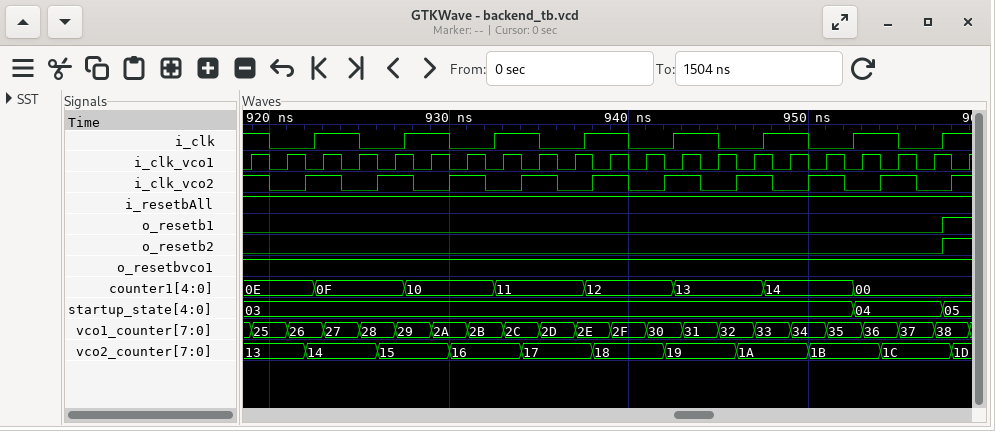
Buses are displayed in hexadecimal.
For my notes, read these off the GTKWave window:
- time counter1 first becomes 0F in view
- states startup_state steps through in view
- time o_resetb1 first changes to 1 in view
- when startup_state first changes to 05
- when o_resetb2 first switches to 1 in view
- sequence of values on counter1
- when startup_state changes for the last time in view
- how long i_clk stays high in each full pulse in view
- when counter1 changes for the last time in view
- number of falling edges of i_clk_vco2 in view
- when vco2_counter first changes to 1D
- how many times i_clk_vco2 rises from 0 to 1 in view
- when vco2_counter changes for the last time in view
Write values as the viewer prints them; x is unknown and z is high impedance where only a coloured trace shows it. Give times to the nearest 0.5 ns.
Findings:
922.5 ns
03, 04, 05
957.5 ns
957.5 ns
957.5 ns
0E, 0F, 10, 11, 12, 13, 14, 00
957.5 ns
2.5 ns, 2.5 ns, 2.5 ns, 2.5 ns, 2.5 ns, 2.5 ns, 2.5 ns
952.5 ns
10
958 ns
10
958 ns
